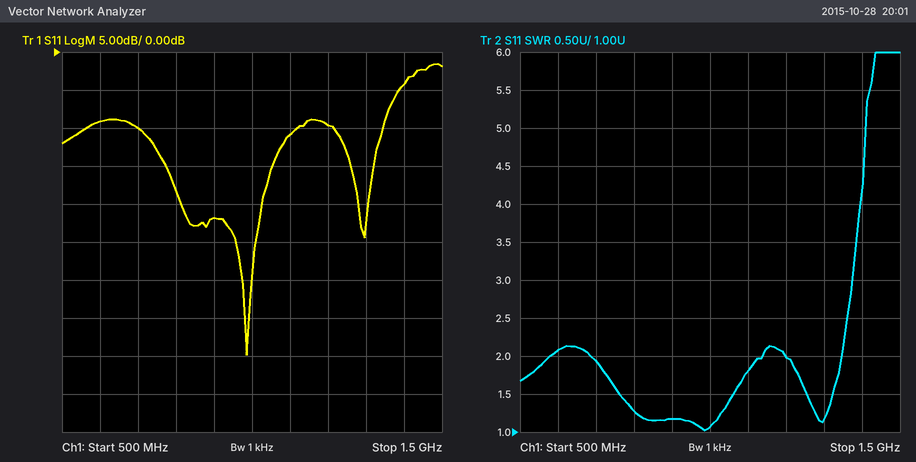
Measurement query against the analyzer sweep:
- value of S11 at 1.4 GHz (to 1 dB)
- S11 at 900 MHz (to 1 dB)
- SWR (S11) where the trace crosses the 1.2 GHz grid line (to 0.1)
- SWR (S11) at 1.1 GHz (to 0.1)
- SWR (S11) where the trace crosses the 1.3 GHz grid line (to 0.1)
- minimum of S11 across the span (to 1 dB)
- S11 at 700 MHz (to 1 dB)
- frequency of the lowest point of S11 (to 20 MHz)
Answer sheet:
-4 dB
-22 dB
2.0
1.8
1.2
-40 dB
-10 dB
980 MHz
